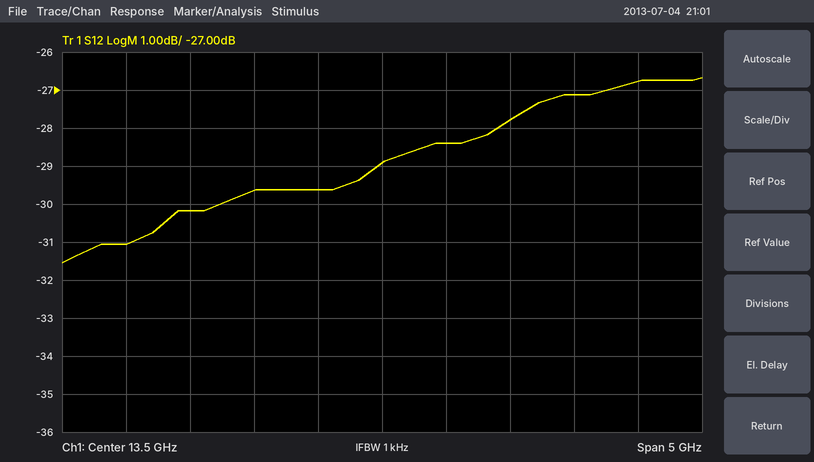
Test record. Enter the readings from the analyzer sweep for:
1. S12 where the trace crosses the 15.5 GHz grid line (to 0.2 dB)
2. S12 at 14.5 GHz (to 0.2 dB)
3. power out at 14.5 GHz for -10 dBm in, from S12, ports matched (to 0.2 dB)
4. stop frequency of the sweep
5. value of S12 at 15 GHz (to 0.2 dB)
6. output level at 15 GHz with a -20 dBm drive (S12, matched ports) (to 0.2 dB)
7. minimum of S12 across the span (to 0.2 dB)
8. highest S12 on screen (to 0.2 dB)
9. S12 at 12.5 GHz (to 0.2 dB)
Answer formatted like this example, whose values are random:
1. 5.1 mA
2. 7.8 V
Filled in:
1. -26.8 dB
2. -27.8 dB
3. -37.8 dBm
4. 16 GHz
5. -27.2 dB
6. -47.2 dBm
7. -31.6 dB
8. -26.6 dB
9. -29.6 dB
